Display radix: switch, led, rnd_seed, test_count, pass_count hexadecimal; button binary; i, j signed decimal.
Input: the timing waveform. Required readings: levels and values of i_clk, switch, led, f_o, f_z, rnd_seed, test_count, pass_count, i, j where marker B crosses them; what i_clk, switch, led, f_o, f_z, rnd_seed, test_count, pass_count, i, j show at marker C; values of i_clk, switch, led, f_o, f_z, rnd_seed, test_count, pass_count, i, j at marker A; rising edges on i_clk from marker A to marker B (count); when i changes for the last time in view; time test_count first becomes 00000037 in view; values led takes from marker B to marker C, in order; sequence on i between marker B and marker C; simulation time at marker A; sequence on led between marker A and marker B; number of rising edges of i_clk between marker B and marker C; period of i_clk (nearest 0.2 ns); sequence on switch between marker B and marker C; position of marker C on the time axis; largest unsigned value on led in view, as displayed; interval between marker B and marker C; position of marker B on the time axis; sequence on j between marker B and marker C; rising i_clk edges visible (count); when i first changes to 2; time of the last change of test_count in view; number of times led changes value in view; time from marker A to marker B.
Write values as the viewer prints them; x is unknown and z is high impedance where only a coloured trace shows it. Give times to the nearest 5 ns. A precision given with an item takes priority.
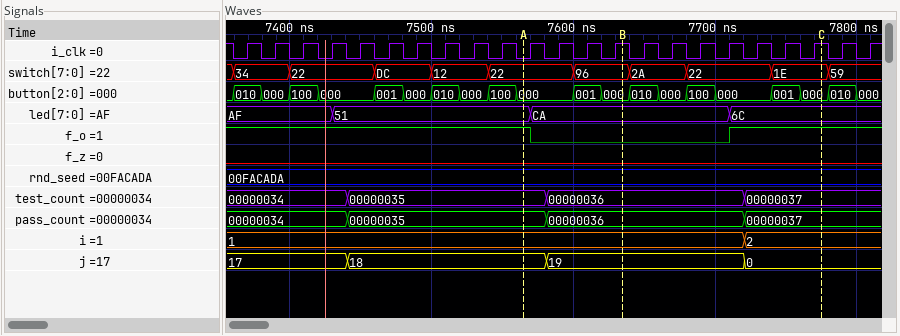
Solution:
i_clk=1, switch=96, led=CA, f_o=0, f_z=0, rnd_seed=00FACADA, test_count=00000036, pass_count=00000036, i=1, j=19
i_clk=1, switch=1E, led=6C, f_o=1, f_z=0, rnd_seed=00FACADA, test_count=00000037, pass_count=00000037, i=2, j=0
i_clk=0, switch=22, led=51, f_o=1, f_z=0, rnd_seed=00FACADA, test_count=00000035, pass_count=00000035, i=1, j=18
4
7720 ns
7720 ns
CA, 6C
1, 2
7565 ns
51, CA
7
20 ns
96, 2A, 22, 1E
7775 ns
CA
140 ns
7635 ns
19, 0
23
7720 ns
7720 ns
3
70 ns
